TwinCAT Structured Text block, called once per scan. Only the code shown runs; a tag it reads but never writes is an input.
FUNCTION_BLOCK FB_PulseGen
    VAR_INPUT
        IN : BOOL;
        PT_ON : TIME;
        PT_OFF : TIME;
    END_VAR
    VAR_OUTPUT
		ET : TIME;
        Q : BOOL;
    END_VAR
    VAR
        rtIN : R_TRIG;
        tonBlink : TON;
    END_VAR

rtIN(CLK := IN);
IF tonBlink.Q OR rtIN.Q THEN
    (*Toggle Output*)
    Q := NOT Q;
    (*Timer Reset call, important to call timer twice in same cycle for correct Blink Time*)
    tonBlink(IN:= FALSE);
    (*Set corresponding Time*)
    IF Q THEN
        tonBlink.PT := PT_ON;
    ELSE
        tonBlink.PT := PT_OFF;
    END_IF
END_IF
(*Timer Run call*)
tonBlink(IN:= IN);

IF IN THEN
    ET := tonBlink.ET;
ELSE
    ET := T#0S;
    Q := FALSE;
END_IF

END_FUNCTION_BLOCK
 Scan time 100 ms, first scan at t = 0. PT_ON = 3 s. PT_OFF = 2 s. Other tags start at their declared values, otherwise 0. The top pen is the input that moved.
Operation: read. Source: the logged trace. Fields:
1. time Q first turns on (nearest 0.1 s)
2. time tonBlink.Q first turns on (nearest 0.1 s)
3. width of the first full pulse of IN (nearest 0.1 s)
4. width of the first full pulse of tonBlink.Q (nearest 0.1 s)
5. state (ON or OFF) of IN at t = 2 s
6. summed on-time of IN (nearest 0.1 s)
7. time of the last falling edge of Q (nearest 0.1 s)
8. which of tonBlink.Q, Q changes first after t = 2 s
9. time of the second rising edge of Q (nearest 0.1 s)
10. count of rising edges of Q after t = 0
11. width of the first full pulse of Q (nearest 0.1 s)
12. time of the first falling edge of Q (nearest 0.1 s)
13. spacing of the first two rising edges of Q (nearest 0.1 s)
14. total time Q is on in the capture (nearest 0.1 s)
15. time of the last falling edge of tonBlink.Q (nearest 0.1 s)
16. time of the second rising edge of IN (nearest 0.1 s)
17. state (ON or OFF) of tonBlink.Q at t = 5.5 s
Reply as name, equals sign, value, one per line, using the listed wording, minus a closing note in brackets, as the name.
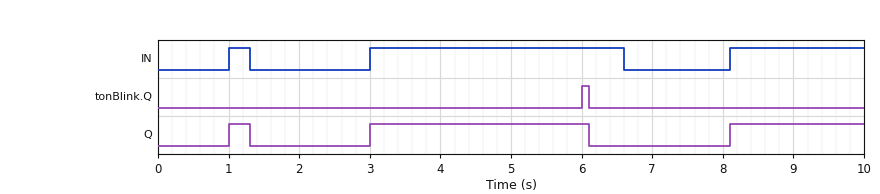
time Q first turns on = 1.0 s
time tonBlink.Q first turns on = 6.0 s
width of the first full pulse of IN = 0.3 s
width of the first full pulse of tonBlink.Q = 0.1 s
state (ON or OFF) of IN at t = 2 s = OFF
summed on-time of IN = 5.8 s
time of the last falling edge of Q = 6.1 s
which of tonBlink.Q, Q changes first after t = 2 s = Q
time of the second rising edge of Q = 3.0 s
count of rising edges of Q after t = 0 = 3
width of the first full pulse of Q = 0.3 s
time of the first falling edge of Q = 1.3 s
spacing of the first two rising edges of Q = 2.0 s
total time Q is on in the capture = 5.3 s
time of the last falling edge of tonBlink.Q = 6.1 s
time of the second rising edge of IN = 3.0 s
state (ON or OFF) of tonBlink.Q at t = 5.5 s = OFF
